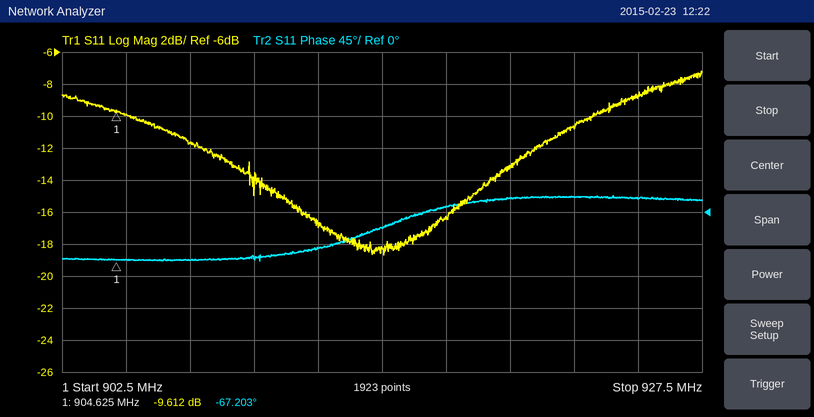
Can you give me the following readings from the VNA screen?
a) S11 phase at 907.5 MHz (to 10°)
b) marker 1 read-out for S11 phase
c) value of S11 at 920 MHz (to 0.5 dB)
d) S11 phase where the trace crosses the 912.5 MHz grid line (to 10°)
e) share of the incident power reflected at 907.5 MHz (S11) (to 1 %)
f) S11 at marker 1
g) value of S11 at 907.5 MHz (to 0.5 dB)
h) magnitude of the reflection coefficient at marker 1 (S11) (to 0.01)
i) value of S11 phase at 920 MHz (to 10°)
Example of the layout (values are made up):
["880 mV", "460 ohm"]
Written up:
["-70°", "-67.203°", "-13.0 dB", "-50°", "7 %", "-9.612 dB", "-11.5 dB", "0.33", "20°"]
